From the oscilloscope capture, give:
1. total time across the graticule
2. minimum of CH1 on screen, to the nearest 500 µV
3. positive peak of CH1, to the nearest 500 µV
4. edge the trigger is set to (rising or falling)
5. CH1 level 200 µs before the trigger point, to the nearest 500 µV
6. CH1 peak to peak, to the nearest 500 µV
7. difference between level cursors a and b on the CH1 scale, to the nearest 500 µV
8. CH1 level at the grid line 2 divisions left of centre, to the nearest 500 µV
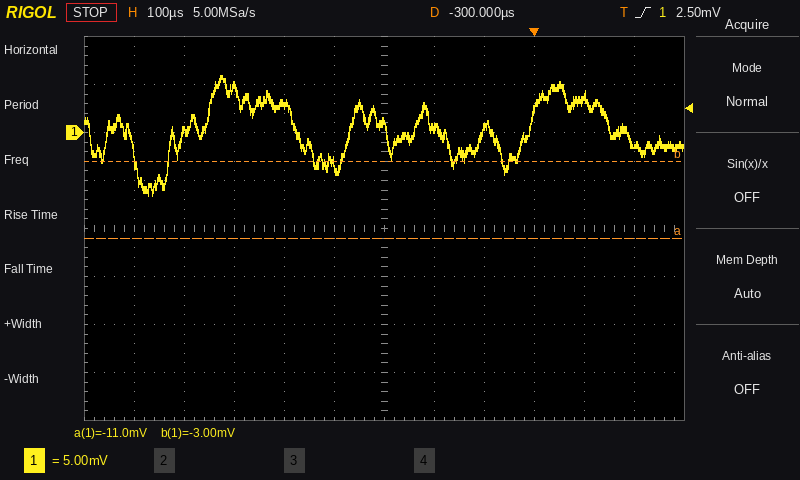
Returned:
1.2 ms
-6.5 mV
6.0 mV
rising
500 µV
12.5 mV
8.0 mV
3.0 mV
